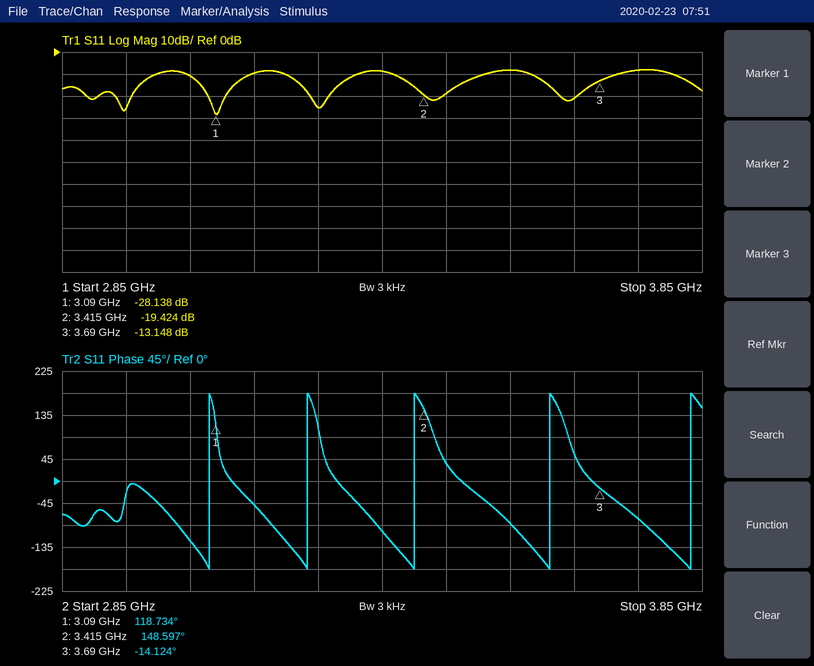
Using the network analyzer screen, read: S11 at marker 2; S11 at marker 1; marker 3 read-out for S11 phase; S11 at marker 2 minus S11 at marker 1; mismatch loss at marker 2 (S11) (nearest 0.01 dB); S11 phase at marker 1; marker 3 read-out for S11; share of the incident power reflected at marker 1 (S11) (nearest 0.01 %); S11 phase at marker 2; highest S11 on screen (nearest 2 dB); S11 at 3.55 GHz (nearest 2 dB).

-19.424 dB
-28.138 dB
-14.124°
8.714 dB
0.05 dB
118.734°
-13.148 dB
0.15 %
148.597°
-8 dB
-8 dB
